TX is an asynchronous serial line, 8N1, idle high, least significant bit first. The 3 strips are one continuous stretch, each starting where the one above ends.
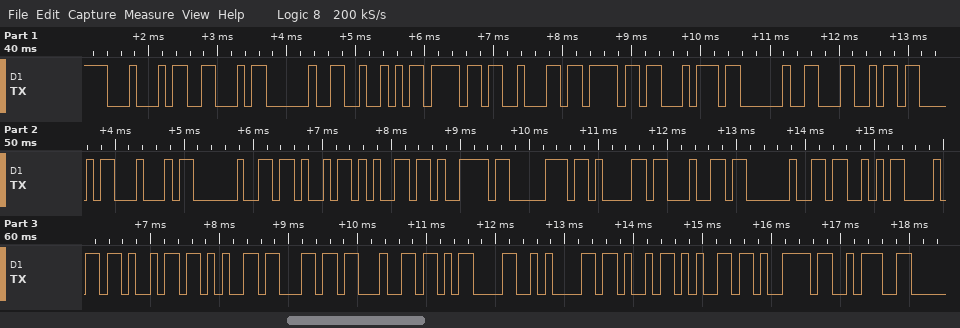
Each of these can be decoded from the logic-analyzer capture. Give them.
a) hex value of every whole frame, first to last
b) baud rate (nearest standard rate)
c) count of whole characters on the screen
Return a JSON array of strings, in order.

["44 46 20 52 6F 62 6F 74 20 4C 43 44 20 4B 65 79 70 61 64 20 53 68 69 65 6C 64 0D 0A 4B 65 79 3A", "9600 baud", "32"]
